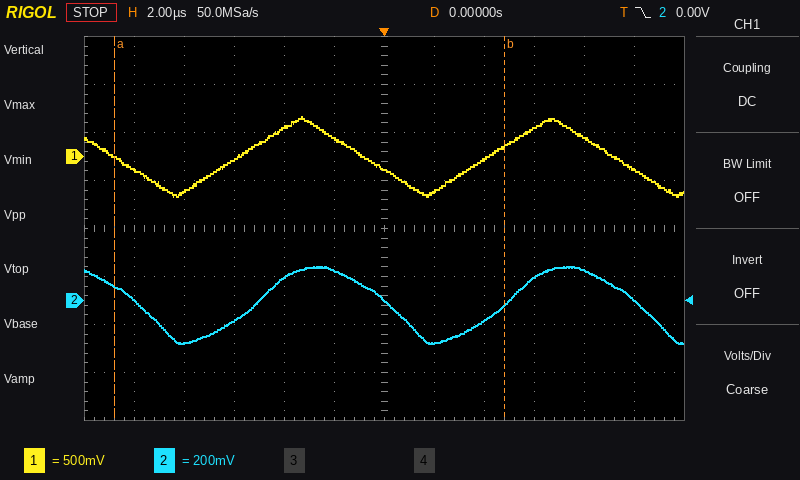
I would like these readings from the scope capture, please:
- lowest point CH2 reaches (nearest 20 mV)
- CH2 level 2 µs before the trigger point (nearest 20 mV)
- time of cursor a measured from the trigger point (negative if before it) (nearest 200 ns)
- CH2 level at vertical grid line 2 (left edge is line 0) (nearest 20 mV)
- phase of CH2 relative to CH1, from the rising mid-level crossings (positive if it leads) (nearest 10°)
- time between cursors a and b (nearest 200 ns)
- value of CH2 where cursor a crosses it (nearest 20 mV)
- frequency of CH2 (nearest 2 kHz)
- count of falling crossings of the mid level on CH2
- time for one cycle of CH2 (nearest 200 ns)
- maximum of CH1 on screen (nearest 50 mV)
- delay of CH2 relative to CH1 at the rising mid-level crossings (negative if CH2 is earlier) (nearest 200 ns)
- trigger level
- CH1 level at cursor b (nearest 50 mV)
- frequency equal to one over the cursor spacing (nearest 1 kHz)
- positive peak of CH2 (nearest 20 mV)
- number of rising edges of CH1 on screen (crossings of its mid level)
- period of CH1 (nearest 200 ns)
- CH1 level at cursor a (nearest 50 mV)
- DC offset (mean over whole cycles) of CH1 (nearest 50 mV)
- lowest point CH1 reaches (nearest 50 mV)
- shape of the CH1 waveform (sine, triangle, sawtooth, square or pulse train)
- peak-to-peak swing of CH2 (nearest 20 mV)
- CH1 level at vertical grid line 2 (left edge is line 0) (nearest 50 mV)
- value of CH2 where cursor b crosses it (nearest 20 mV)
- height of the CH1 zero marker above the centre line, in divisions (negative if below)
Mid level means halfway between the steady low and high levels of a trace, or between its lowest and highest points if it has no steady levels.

-180 mV
120 mV
-10.8 µs
-180 mV
-20°
15.6 µs
60 mV
100 kHz
3
10.0 µs
400 mV
+600 ns
0.00 V
100 mV
64 kHz
140 mV
2
10.0 µs
0 mV
0 mV
-400 mV
triangle
320 mV
-350 mV
-20 mV
+1.5 div
